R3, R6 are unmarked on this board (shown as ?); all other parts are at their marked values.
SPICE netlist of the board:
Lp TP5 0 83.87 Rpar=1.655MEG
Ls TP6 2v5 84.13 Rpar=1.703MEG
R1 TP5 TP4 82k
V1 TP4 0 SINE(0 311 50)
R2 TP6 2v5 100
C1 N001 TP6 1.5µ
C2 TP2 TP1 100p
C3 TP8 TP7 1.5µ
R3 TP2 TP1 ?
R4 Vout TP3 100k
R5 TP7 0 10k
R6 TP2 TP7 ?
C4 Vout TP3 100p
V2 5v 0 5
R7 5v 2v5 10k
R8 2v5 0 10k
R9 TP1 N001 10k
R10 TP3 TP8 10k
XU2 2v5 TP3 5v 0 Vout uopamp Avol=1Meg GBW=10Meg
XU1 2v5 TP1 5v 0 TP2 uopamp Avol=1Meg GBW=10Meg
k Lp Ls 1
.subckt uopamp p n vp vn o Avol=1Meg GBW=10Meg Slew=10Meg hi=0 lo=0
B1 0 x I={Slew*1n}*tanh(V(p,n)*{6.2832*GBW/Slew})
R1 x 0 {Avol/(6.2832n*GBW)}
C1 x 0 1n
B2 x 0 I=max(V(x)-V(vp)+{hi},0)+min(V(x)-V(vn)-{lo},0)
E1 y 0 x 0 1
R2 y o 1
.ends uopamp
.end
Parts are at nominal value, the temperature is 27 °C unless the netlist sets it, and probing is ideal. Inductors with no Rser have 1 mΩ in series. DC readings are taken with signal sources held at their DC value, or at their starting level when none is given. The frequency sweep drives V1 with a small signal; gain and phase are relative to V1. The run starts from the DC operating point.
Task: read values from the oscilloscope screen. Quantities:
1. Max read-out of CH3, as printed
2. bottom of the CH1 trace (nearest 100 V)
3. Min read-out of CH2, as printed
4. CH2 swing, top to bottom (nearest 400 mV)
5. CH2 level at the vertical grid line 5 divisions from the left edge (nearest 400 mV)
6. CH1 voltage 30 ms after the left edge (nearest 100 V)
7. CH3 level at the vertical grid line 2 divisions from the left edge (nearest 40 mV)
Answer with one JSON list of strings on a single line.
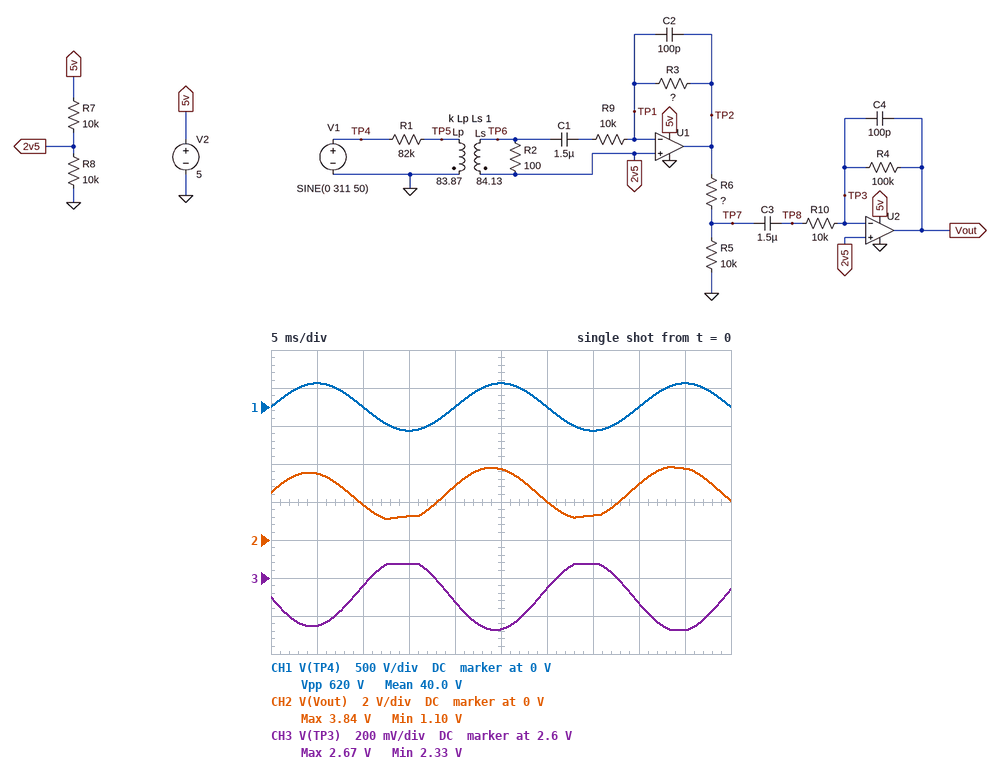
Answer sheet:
["2.67 V", "-300 V", "1.10 V", "2.8 V", "3.6 V", "0 V", "2.56 V"]
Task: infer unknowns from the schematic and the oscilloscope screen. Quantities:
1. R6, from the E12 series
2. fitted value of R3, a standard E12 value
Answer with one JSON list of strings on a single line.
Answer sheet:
["47 kΩ", "68 kΩ"]
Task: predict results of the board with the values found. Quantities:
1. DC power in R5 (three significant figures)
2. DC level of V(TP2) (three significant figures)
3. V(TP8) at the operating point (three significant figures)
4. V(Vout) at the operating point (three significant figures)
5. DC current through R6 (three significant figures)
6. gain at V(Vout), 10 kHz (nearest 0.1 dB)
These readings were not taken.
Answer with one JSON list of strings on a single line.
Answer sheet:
["19.2 µW", "2.50 V", "2.50 V", "2.50 V", "43.9 µA", "-48.2 dB"]
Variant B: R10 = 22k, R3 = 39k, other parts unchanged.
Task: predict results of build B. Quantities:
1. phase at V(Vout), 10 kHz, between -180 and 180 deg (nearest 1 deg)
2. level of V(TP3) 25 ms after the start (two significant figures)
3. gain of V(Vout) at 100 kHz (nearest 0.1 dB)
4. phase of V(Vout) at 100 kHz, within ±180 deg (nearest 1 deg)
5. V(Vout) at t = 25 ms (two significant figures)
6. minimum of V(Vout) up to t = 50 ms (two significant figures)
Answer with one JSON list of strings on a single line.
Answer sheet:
["-105 deg", "2.3 V", "-62.1 dB", "166 deg", "2.6 V", "2.3 V"]
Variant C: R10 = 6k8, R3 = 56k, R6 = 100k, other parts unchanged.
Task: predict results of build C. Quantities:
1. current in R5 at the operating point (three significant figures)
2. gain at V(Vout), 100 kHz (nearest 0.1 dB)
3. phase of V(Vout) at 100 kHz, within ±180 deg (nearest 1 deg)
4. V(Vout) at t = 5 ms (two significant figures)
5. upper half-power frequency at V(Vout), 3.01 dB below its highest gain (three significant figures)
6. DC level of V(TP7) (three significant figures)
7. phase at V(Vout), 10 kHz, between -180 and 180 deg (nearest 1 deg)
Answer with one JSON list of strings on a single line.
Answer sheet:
["22.7 µA", "-60.6 dB", "150 deg", "2.4 V", "57.6 kHz", "227 mV", "-144 deg"]
